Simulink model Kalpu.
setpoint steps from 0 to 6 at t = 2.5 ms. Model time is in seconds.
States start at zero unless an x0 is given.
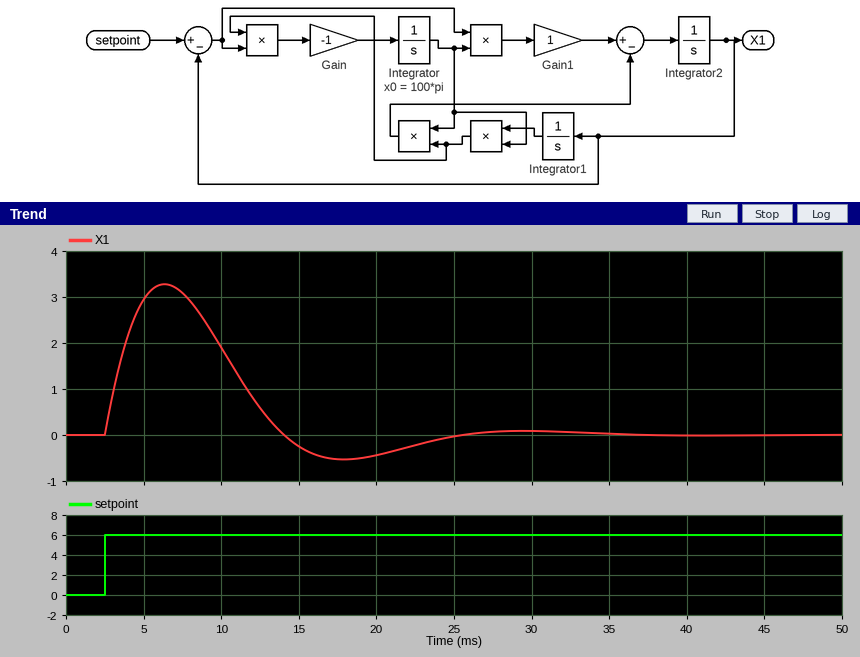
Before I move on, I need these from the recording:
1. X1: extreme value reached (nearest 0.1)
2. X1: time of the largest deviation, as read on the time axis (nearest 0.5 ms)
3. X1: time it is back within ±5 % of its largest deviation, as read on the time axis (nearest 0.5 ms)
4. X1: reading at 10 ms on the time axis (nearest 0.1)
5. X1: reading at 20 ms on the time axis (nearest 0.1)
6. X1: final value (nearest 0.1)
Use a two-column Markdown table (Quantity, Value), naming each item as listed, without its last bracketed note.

| Quantity | Value |
|---|---|
| X1: extreme value reached | 3.3 |
| X1: time of the largest deviation, as read on the time axis | 6.5 ms |
| X1: time it is back within ±5 % of its largest deviation, as read on the time axis | 23.0 ms |
| X1: reading at 10 ms on the time axis | 1.9 |
| X1: reading at 20 ms on the time axis | -0.4 |
| X1: final value | 0.0 |
